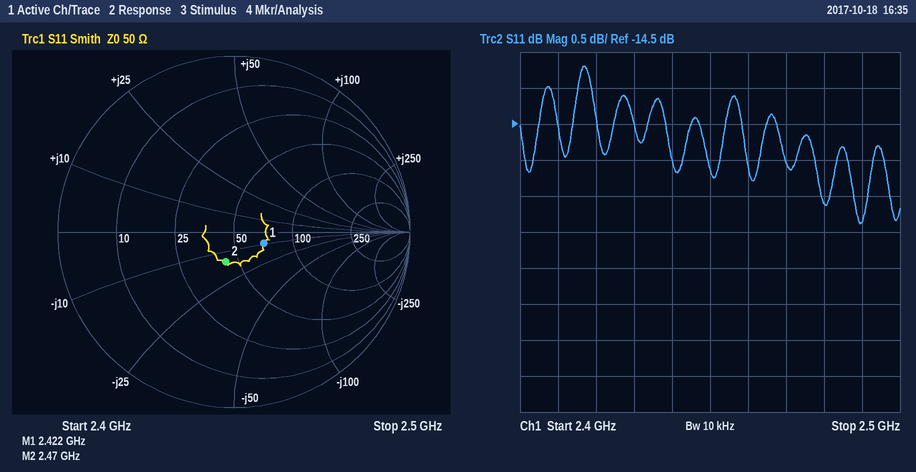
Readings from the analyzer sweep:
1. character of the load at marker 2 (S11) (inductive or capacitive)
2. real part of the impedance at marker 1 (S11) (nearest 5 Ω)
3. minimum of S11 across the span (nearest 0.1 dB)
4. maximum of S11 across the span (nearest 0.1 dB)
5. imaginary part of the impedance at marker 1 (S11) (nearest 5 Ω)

capacitive
70 Ω
-15.9 dB
-13.7 dB
-10 Ω
